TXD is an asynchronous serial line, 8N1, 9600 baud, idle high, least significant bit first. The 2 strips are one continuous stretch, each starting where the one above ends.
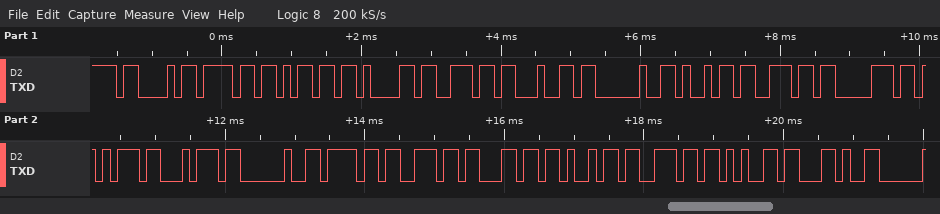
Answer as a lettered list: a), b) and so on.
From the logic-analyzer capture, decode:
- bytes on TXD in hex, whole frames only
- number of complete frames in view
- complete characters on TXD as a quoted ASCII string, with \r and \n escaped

a) 43 6F 6D 61 6E 64 20 69 6E 70 75 74 20 6F 6E 6C 69 6E 65 2C
b) 20
c) "Comand input online,"
